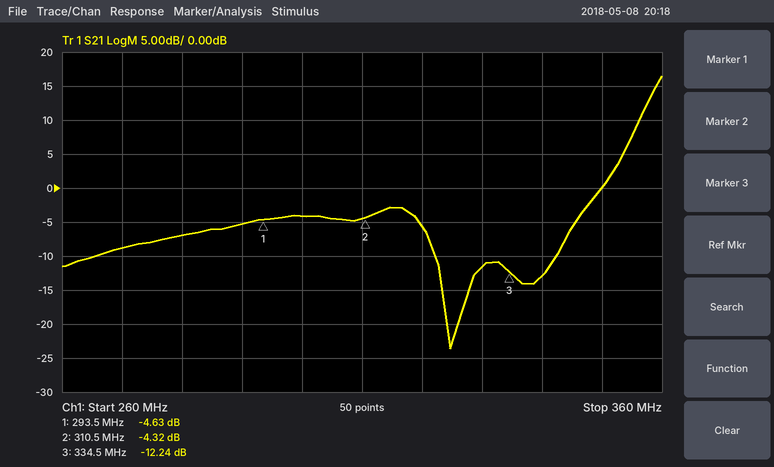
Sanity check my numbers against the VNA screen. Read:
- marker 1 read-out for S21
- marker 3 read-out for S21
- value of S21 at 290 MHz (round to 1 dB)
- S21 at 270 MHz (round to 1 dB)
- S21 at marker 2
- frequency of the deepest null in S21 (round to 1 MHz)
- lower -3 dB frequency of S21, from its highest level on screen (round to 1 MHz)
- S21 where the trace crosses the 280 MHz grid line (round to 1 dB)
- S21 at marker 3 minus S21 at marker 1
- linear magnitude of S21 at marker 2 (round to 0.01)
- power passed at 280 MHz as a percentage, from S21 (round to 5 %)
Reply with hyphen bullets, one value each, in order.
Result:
- -4.63 dB
- -12.24 dB
- -5 dB
- -9 dB
- -4.32 dB
- 325 MHz
- 358 MHz
- -7 dB
- -7.61 dB
- 0.61
- 20 %
